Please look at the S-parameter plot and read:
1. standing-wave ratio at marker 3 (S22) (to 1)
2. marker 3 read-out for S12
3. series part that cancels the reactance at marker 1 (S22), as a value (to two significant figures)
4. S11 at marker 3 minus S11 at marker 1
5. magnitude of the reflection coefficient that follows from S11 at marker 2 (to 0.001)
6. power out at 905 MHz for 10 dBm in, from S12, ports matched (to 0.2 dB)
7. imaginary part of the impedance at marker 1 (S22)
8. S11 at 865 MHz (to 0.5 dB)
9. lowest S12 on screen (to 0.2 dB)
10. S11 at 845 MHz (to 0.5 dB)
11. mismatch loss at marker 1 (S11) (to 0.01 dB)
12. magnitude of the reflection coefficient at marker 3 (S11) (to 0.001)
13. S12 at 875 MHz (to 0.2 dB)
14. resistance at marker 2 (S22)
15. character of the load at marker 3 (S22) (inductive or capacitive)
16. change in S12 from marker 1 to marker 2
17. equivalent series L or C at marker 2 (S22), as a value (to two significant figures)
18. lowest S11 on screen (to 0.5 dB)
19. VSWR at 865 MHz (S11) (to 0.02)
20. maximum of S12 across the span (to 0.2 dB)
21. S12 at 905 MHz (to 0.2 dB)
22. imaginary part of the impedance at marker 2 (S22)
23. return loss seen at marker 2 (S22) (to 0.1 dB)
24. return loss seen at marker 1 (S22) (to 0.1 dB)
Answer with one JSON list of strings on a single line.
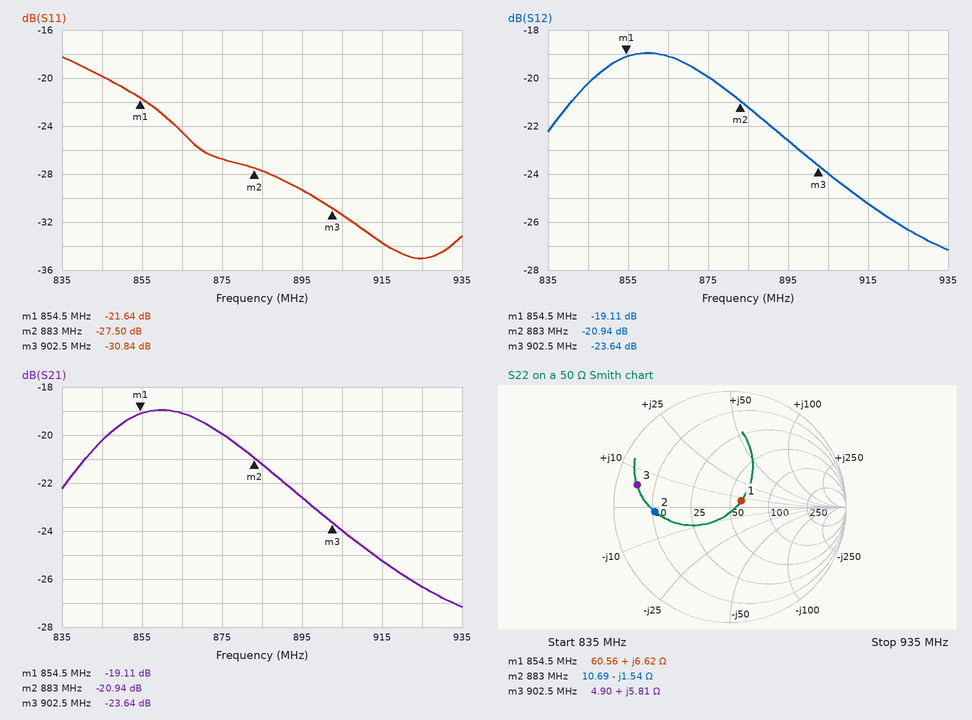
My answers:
["10", "-23.64 dB", "28 pF", "-9.20 dB", "0.042", "-14.0 dBm", "+6.62 Ω", "-24.5 dB", "-27.2 dB", "-20.0 dB", "0.03 dB", "0.029", "-20.0 dB", "10.69 Ω", "inductive", "-1.83 dB", "120 pF", "-35.0 dB", "1.12", "-19.0 dB", "-24.0 dB", "-1.54 Ω", "3.8 dB", "19.0 dB"]
